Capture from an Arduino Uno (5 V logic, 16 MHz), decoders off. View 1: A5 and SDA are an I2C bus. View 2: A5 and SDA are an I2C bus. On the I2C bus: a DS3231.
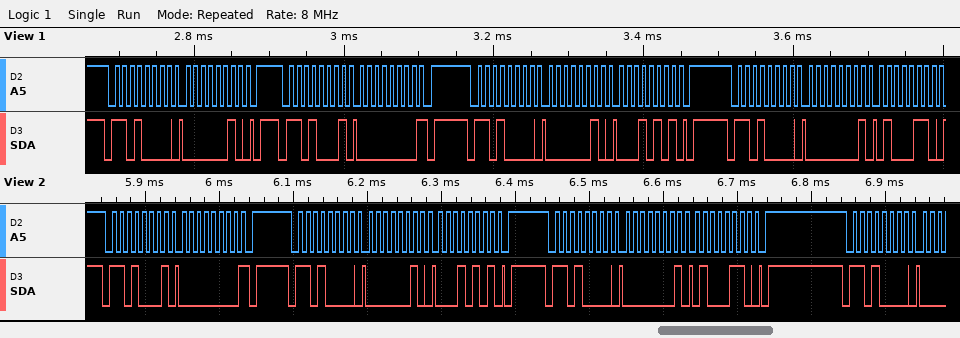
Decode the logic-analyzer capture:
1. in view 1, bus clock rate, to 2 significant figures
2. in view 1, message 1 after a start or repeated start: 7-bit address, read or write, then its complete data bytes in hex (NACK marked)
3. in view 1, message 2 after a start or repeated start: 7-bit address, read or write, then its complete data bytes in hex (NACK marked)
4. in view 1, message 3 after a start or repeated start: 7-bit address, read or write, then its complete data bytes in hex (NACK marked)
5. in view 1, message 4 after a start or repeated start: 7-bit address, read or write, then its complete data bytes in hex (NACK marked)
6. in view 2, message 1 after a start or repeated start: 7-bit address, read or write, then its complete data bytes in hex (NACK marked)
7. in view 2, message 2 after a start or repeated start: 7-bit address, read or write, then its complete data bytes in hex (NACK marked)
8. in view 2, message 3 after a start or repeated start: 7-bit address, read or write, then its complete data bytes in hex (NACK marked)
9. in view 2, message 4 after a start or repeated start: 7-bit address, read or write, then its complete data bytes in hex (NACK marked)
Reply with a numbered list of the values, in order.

1. 100 kHz
2. 0x68 write: 02
3. 0x68 read: 00 NACK
4. 0x68 write: 02 15
5. 0x68 write: 01 46
6. 0x68 read: 00 NACK
7. 0x68 write: 02 15
8. 0x68 write: 01 46
9. 0x68 write
